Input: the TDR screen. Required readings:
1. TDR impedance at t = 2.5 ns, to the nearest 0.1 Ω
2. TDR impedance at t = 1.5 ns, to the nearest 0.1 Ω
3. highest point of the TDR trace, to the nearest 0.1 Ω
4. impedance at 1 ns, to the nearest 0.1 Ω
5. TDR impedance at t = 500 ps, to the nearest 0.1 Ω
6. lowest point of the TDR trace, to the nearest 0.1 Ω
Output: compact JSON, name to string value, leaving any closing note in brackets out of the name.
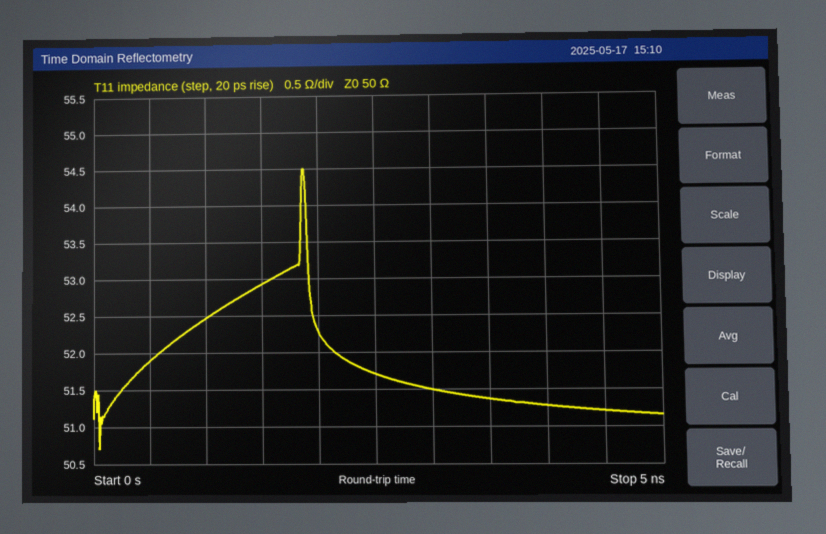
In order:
{"TDR impedance at t = 2.5 ns, to the nearest 0.1 Ω": "51.7 Ω", "TDR impedance at t = 1.5 ns, to the nearest 0.1 Ω": "52.9 Ω", "highest point of the TDR trace, to the nearest 0.1 Ω": "54.5 Ω", "impedance at 1 ns, to the nearest 0.1 Ω": "52.5 Ω", "TDR impedance at t = 500 ps, to the nearest 0.1 Ω": "51.9 Ω", "lowest point of the TDR trace, to the nearest 0.1 Ω": "50.7 Ω"}
